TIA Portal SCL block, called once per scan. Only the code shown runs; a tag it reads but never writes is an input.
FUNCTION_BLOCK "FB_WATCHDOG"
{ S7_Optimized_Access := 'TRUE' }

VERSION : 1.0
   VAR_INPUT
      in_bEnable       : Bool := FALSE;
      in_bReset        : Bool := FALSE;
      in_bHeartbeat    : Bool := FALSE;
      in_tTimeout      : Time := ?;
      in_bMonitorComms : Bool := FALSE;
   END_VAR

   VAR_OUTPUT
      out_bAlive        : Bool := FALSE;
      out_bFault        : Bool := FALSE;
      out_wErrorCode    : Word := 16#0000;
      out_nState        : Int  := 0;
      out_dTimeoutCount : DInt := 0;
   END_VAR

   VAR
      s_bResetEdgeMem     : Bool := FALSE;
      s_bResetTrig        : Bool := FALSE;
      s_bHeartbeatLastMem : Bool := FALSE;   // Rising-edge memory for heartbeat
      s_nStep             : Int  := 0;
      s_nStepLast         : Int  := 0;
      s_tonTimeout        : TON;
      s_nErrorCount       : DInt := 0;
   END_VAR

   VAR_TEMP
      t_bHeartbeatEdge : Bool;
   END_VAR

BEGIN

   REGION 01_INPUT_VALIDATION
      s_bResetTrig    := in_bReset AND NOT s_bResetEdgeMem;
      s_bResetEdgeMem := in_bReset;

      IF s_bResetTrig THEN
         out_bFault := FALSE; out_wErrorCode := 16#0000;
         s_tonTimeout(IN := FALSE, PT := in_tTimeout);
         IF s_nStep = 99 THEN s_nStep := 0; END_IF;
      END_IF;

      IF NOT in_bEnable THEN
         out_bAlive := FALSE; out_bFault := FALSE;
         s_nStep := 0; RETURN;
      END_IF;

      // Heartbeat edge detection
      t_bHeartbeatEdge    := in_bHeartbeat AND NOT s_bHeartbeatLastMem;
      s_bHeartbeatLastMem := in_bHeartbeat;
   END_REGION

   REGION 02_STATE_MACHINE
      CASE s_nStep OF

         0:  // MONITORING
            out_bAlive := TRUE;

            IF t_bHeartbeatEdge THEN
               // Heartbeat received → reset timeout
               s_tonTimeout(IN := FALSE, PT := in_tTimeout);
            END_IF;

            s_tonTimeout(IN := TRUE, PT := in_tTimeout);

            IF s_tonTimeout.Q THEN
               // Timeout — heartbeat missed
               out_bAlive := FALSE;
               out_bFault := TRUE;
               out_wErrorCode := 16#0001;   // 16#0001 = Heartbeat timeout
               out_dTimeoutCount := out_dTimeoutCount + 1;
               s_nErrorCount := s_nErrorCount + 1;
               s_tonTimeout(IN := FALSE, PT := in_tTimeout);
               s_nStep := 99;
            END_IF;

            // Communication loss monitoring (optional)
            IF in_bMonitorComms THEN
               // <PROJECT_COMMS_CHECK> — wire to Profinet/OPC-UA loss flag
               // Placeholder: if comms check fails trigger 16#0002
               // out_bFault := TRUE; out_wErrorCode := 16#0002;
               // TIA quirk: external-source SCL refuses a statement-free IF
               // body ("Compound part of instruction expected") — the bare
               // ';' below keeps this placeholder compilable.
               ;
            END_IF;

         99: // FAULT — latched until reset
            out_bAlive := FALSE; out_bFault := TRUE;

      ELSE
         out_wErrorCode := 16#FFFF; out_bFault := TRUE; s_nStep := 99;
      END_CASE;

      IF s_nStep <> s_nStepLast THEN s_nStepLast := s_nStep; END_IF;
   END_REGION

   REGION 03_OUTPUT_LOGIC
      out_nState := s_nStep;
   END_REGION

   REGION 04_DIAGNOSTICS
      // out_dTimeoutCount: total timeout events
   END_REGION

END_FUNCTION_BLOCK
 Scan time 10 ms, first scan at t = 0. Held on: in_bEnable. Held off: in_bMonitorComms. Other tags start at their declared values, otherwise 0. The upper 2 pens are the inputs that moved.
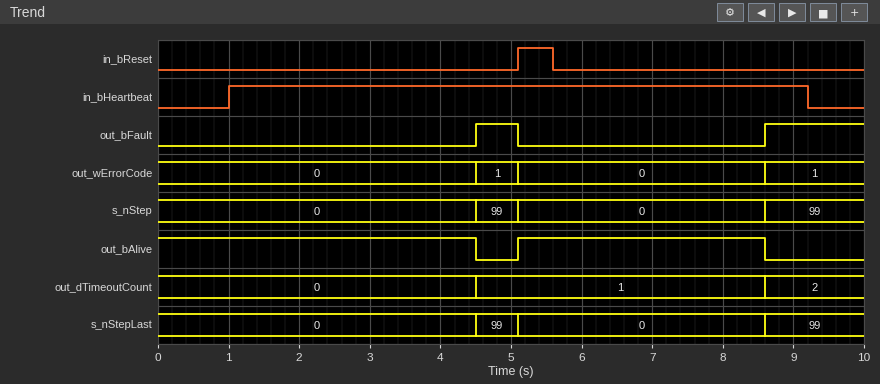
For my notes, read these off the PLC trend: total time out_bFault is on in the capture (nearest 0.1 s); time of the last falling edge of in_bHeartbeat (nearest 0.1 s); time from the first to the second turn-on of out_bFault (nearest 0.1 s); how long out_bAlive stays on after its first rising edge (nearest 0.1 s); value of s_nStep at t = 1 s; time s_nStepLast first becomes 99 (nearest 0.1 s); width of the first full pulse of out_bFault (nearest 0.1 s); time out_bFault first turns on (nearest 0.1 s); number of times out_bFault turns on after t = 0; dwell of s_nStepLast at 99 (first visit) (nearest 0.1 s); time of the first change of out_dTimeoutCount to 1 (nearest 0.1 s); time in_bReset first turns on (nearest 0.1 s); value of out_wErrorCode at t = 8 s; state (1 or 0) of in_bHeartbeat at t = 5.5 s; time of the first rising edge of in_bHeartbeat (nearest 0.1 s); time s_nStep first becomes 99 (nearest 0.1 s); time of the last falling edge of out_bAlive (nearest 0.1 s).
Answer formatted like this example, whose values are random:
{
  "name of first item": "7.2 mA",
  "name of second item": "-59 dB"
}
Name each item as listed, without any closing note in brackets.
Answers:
{
  "total time out_bFault is on in the capture": "2.0 s",
  "time of the last falling edge of in_bHeartbeat": "9.2 s",
  "time from the first to the second turn-on of out_bFault": "4.1 s",
  "how long out_bAlive stays on after its first rising edge": "3.5 s",
  "value of s_nStep at t = 1 s": "0",
  "time s_nStepLast first becomes 99": "4.5 s",
  "width of the first full pulse of out_bFault": "0.6 s",
  "time out_bFault first turns on": "4.5 s",
  "number of times out_bFault turns on after t = 0": "2",
  "dwell of s_nStepLast at 99 (first visit)": "0.6 s",
  "time of the first change of out_dTimeoutCount to 1": "4.5 s",
  "time in_bReset first turns on": "5.1 s",
  "value of out_wErrorCode at t = 8 s": "0",
  "state (1 or 0) of in_bHeartbeat at t = 5.5 s": "1",
  "time of the first rising edge of in_bHeartbeat": "1.0 s",
  "time s_nStep first becomes 99": "4.5 s",
  "time of the last falling edge of out_bAlive": "8.6 s"
}
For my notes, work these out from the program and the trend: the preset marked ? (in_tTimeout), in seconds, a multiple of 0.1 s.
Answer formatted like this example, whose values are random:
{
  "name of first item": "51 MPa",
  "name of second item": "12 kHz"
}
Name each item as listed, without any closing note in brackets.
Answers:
{
  "the preset marked ? (in_tTimeout), in seconds, a multiple of 0.1 s": "3.5 s"
}
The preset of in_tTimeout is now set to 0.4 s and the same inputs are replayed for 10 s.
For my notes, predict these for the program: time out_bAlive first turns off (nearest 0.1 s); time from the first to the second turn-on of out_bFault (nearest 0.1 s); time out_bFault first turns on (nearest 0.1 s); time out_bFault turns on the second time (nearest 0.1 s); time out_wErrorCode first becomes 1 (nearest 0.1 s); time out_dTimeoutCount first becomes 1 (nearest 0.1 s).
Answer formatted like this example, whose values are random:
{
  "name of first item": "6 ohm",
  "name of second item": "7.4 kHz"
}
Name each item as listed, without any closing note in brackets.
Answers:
{
  "time out_bAlive first turns off": "0.4 s",
  "time from the first to the second turn-on of out_bFault": "5.1 s",
  "time out_bFault first turns on": "0.4 s",
  "time out_bFault turns on the second time": "5.5 s",
  "time out_wErrorCode first becomes 1": "0.4 s",
  "time out_dTimeoutCount first becomes 1": "0.4 s"
}
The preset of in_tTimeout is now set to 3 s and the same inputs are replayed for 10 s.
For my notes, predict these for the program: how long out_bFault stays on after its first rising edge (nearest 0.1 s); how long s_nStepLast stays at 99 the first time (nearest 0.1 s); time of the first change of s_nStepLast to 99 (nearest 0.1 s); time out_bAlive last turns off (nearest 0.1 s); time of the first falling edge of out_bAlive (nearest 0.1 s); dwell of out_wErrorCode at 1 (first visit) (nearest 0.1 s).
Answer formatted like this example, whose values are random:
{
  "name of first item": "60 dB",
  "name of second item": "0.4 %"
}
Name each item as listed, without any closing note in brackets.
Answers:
{
  "how long out_bFault stays on after its first rising edge": "1.1 s",
  "how long s_nStepLast stays at 99 the first time": "1.1 s",
  "time of the first change of s_nStepLast to 99": "4.0 s",
  "time out_bAlive last turns off": "8.1 s",
  "time of the first falling edge of out_bAlive": "4.0 s",
  "dwell of out_wErrorCode at 1 (first visit)": "1.1 s"
}
